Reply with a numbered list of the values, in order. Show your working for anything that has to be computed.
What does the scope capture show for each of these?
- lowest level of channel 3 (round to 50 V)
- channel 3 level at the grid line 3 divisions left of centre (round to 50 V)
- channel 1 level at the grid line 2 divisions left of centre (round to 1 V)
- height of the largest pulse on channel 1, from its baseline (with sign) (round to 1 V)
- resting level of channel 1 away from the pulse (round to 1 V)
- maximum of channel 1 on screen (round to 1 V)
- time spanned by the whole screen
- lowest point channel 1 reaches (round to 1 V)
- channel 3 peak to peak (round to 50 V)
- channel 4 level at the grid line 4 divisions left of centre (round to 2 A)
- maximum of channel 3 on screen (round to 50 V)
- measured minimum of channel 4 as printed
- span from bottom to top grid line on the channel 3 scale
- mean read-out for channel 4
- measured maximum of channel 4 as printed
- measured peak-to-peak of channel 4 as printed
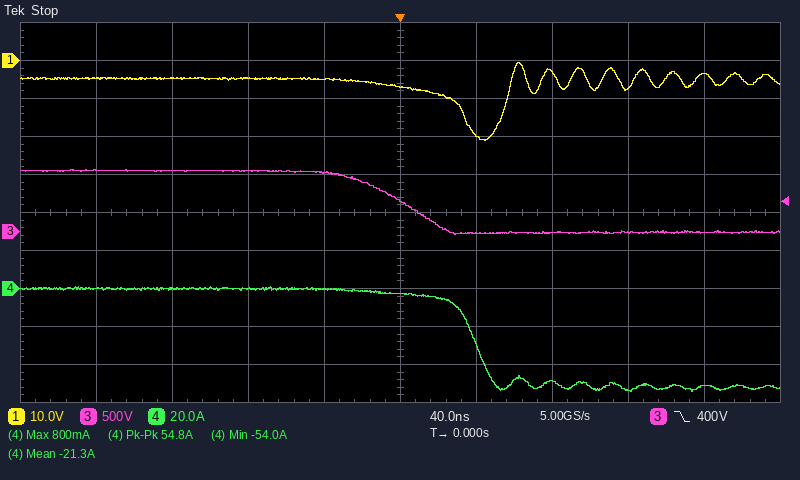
1. -50 V
2. 800 V
3. -5 V
4. -21 V − (-5 V) = -16 V
5. -5 V
6. -1 V
7. 400 ns
8. -21 V
9. 800 V − (-50 V) = 850 V
10. 0 A
11. 800 V
12. -54.0 A
13. 5 kV
14. -21.3 A
15. 800 mA
16. 54.8 A
